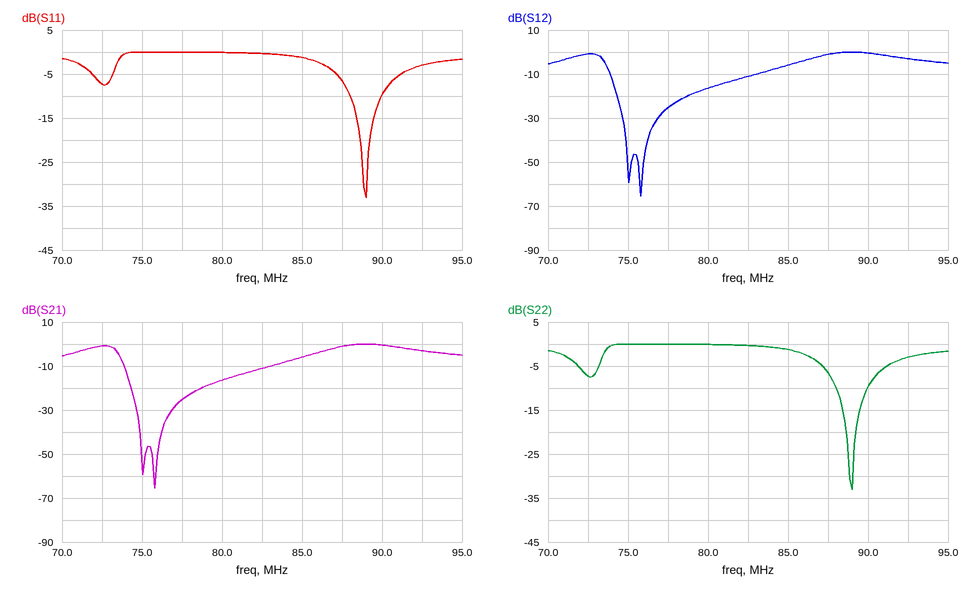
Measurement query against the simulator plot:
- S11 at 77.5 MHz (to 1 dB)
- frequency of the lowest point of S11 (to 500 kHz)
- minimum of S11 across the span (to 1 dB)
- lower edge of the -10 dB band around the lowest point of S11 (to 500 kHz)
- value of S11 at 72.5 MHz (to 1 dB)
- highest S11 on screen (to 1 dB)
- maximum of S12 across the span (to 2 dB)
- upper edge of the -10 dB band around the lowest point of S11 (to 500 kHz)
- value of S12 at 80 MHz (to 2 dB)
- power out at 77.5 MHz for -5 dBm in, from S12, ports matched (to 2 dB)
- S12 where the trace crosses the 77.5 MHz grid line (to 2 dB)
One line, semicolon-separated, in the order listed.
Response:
0 dB; 89.0 MHz; -33 dB; 88.0 MHz; -7 dB; 0 dB; 0 dB; 90.0 MHz; -16 dB; -30 dBm; -26 dB
